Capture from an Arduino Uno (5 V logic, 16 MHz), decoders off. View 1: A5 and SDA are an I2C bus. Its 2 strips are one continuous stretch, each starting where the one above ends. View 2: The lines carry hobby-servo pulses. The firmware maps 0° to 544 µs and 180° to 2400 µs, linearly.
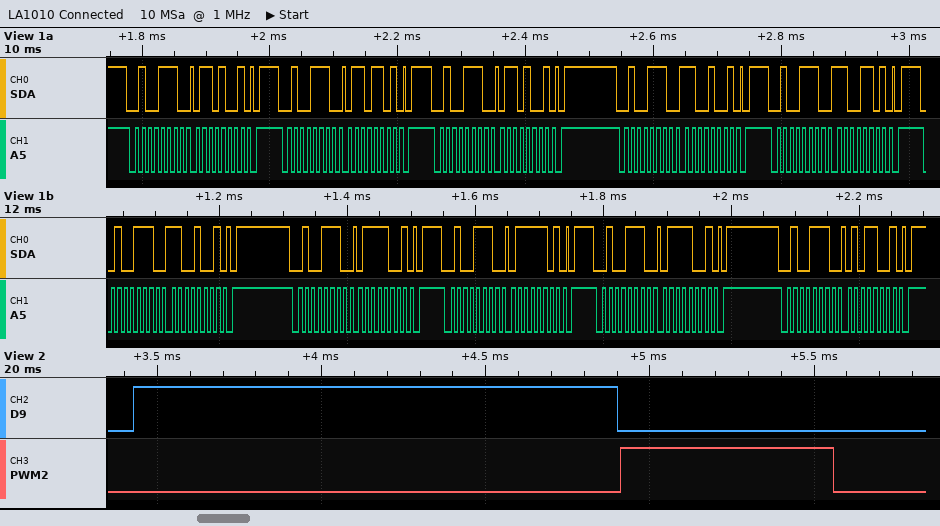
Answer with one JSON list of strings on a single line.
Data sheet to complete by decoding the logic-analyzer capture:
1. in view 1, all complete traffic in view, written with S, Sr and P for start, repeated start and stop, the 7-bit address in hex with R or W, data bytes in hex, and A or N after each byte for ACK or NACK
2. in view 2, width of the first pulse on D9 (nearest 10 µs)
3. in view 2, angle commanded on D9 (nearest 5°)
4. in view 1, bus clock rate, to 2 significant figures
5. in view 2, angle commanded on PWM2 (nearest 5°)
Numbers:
["S 27W A 69 A P S 27W A 6D A P S 27W A 69 A P S 27W A C9 A P S 27W A CD A P S 27W A C9 A P S 27W A 79 A P S 27W A 7D A P S 27W A 79 A P S 27W A 59 A P", "1470 µs", "90°", "100 kHz", "10°"]
